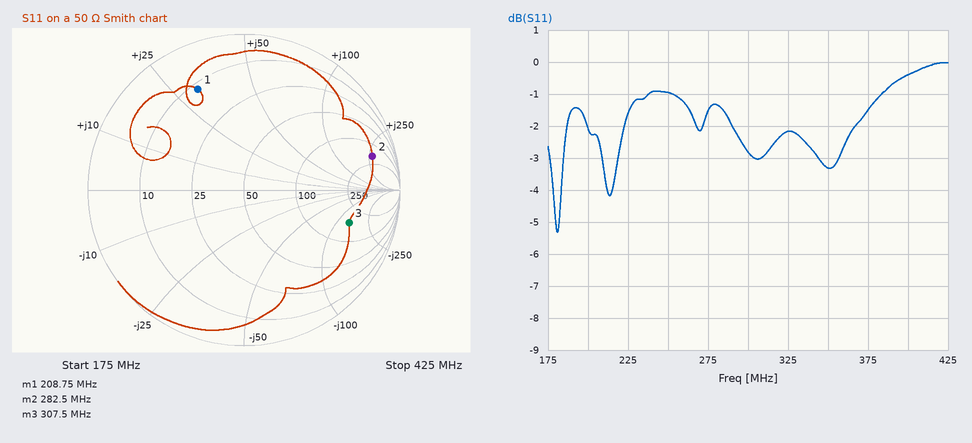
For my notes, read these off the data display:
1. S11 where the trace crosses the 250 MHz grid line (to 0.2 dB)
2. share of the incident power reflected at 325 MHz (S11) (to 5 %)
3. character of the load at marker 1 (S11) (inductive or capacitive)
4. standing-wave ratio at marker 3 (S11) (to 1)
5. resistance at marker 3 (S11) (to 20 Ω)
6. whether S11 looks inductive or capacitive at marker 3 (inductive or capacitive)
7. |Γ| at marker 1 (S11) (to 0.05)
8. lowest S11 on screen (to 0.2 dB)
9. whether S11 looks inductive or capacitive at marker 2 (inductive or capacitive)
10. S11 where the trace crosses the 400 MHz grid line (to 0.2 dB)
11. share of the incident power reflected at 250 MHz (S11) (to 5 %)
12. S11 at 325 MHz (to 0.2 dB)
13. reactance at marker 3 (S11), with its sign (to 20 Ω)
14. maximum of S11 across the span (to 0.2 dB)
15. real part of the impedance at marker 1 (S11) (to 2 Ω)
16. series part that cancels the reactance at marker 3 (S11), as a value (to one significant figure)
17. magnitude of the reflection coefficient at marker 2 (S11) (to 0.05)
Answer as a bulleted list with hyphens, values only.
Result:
- -1.0 dB
- 60 %
- inductive
- 6
- 160 Ω
- capacitive
- 0.70
- -5.4 dB
- inductive
- -0.4 dB
- 80 %
- -2.2 dB
- -140 Ω
- 0.0 dB
- 12 Ω
- 70 nH
- 0.85
